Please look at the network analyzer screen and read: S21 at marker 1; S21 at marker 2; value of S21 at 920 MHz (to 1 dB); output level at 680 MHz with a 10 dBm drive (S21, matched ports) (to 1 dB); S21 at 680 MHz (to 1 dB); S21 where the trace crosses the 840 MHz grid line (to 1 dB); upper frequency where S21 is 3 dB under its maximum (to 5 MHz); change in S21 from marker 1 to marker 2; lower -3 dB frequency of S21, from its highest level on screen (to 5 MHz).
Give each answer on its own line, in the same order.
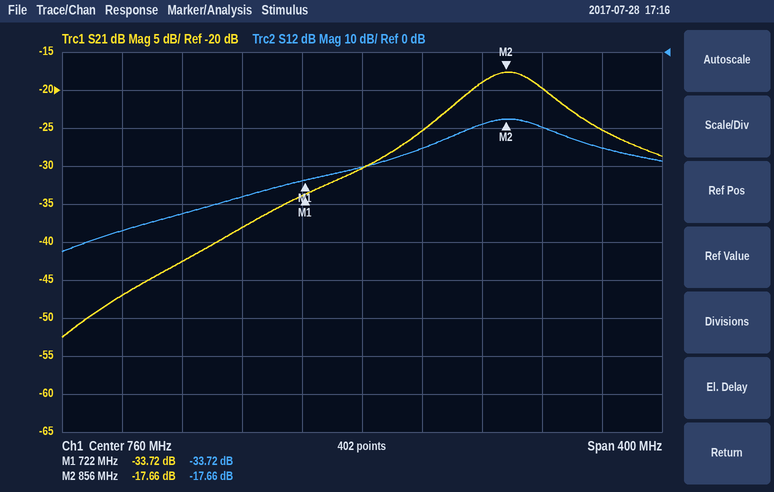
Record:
-33.72 dB
-17.66 dB
-25 dB
-28 dBm
-38 dB
-19 dB
885 MHz
16.06 dB
830 MHz
